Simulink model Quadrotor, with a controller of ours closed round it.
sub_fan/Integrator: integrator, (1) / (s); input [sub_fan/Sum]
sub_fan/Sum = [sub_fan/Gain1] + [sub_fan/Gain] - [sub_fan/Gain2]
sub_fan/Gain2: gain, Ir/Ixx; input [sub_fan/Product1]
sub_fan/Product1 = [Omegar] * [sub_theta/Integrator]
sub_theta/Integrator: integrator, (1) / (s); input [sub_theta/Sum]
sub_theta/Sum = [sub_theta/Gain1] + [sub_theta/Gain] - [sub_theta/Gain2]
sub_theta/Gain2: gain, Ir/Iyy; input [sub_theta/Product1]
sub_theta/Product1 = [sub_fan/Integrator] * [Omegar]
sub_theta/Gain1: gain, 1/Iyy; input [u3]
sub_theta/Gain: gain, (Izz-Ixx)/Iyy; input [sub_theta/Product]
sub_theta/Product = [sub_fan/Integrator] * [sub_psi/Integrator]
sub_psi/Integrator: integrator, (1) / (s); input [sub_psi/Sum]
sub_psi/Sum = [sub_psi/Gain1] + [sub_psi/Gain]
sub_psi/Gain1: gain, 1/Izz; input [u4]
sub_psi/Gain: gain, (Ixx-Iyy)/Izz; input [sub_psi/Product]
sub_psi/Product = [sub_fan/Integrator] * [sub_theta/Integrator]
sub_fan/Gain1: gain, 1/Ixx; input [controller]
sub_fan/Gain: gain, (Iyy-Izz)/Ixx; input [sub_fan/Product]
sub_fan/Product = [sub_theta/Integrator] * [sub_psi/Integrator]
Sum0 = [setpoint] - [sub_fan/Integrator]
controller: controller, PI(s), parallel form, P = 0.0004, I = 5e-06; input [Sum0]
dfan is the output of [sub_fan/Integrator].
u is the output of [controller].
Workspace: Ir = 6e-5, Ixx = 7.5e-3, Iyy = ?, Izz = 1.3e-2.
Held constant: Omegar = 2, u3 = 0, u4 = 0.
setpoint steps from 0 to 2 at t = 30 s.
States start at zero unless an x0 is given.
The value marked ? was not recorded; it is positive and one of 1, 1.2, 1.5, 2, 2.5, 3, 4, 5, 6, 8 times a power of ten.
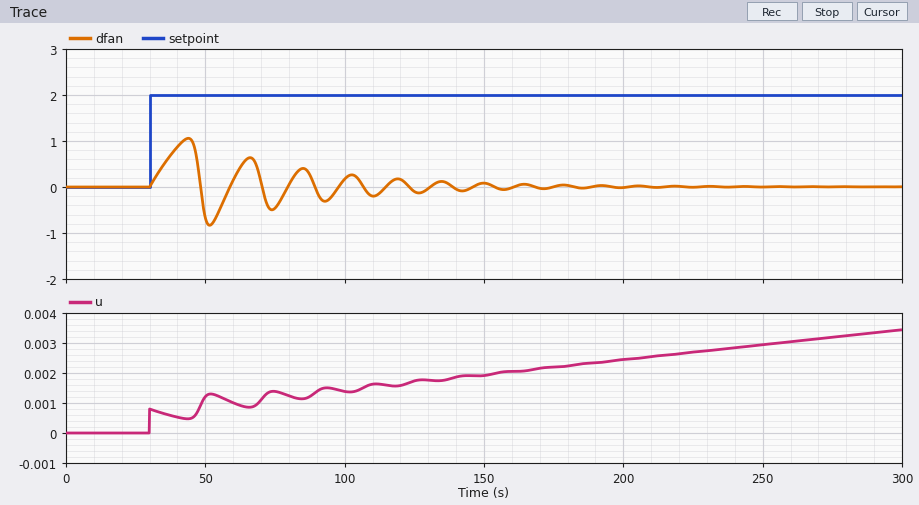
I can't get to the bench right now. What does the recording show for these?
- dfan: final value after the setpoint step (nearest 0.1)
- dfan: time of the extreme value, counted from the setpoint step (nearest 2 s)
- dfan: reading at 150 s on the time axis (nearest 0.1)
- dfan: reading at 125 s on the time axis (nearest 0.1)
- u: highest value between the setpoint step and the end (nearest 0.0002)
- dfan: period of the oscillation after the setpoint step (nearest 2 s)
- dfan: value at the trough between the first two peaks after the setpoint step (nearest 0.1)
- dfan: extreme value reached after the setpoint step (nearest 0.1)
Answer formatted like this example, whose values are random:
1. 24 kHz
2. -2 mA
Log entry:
1. 0.0
2. 14 s
3. 0.1
4. -0.1
5. 0.0034
6. 22 s
7. -0.8
8. 1.1
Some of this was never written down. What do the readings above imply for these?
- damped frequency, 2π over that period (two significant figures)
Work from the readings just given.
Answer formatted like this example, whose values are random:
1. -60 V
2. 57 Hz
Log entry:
1. 0.29 rad/s
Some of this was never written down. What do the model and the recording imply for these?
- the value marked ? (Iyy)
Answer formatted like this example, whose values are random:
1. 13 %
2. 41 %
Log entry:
1. 0.006
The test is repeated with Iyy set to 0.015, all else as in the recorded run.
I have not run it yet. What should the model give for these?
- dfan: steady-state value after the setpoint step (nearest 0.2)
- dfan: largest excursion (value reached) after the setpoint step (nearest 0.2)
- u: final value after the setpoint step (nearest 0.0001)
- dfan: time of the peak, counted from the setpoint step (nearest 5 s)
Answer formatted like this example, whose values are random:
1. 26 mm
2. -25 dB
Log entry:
1. 2.0
2. 2.2
3. 0.0000
4. 75 s
